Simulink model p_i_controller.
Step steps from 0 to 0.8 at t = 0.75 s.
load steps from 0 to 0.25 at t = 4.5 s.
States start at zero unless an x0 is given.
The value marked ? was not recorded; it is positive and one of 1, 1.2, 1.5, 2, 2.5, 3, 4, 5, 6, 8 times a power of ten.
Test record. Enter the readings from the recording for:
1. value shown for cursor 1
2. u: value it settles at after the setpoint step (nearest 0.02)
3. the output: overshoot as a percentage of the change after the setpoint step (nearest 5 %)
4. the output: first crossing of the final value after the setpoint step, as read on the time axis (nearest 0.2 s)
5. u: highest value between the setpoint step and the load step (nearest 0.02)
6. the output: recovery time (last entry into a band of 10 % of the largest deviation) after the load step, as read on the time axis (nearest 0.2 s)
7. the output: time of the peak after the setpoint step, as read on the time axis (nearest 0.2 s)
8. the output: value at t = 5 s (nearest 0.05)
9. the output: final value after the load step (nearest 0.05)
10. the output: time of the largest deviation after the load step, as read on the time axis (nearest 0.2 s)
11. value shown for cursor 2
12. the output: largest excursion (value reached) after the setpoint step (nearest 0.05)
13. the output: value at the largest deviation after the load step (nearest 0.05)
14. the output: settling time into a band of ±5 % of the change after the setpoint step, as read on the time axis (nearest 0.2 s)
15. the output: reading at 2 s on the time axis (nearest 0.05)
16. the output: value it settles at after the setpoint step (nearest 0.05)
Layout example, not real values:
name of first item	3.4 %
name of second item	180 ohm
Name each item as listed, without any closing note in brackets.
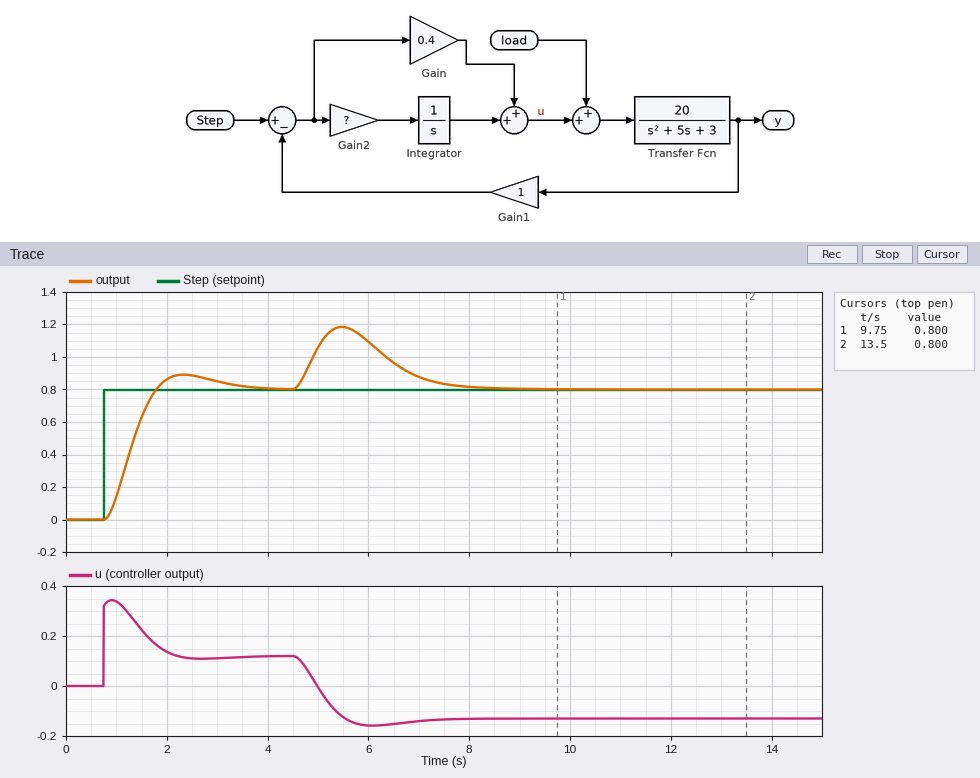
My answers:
value shown for cursor 1	0.800
u: value it settles at after the setpoint step	0.12
the output: overshoot as a percentage of the change after the setpoint step	10 %
the output: first crossing of the final value after the setpoint step, as read on the time axis	1.8 s
u: highest value between the setpoint step and the load step	0.34
the output: recovery time (last entry into a band of 10 % of the largest deviation) after the load step, as read on the time axis	7.4 s
the output: time of the peak after the setpoint step, as read on the time axis	2.4 s
the output: value at t = 5 s	1.05
the output: final value after the load step	0.80
the output: time of the largest deviation after the load step, as read on the time axis	5.4 s
value shown for cursor 2	0.800
the output: largest excursion (value reached) after the setpoint step	0.90
the output: value at the largest deviation after the load step	1.20
the output: settling time into a band of ±5 % of the change after the setpoint step, as read on the time axis	3.2 s
the output: reading at 2 s on the time axis	0.85
the output: value it settles at after the setpoint step	0.80
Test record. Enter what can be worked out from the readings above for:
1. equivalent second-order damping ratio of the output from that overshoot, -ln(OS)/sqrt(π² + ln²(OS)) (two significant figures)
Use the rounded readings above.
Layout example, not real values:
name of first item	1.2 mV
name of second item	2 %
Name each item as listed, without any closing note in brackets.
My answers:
equivalent second-order damping ratio of the output from that overshoot, -ln(OS)/sqrt(π² + ln²(OS))	0.59
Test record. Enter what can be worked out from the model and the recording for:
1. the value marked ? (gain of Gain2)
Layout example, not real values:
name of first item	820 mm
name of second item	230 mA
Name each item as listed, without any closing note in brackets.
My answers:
the value marked ?	0.4
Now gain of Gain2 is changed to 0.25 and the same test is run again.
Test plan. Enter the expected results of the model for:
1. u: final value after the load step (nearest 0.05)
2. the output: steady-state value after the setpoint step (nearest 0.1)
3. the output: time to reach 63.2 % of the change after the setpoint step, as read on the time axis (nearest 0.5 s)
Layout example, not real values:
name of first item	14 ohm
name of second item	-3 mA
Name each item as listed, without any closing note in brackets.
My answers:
u: final value after the load step	-0.15
the output: steady-state value after the setpoint step	0.8
the output: time to reach 63.2 % of the change after the setpoint step, as read on the time axis	1.5 s
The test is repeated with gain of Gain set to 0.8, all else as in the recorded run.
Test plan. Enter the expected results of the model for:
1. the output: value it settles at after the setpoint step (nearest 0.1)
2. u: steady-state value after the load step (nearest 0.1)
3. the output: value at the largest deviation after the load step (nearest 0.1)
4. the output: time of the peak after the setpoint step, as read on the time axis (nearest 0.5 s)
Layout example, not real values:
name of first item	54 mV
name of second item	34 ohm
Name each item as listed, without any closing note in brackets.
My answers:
the output: value it settles at after the setpoint step	0.8
u: steady-state value after the load step	-0.1
the output: value at the largest deviation after the load step	1.1
the output: time of the peak after the setpoint step, as read on the time axis	1.5 s
